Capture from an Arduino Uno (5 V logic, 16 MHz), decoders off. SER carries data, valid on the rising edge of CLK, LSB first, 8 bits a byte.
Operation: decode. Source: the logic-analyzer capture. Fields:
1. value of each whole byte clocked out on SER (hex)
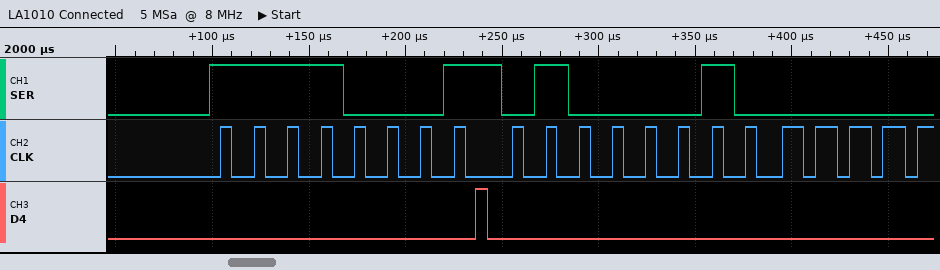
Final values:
0x8F 0x42
